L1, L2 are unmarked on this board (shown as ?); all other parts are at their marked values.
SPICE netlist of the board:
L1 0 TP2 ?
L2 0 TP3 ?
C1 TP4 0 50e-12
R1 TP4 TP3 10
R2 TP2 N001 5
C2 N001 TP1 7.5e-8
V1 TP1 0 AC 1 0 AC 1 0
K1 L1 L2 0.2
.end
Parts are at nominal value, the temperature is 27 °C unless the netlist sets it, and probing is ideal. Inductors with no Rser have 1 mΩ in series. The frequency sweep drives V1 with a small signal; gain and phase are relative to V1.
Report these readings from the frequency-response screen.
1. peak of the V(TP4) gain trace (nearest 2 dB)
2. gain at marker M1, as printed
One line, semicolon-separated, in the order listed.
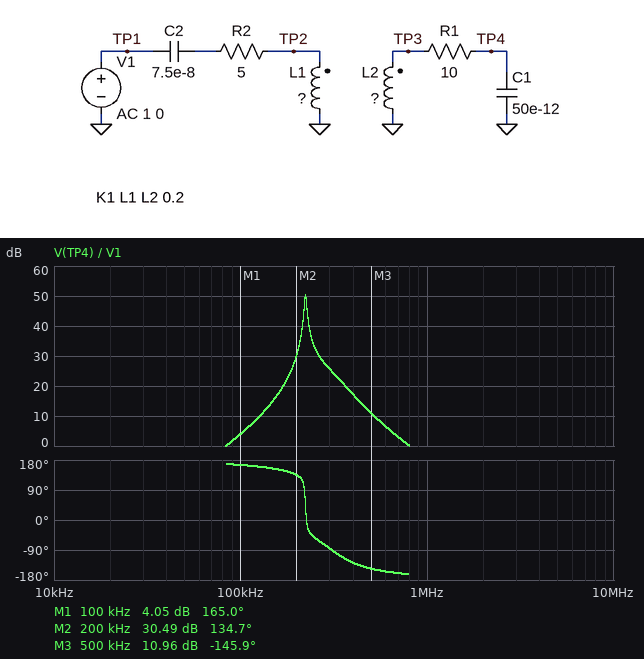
50 dB; 4.05 dB
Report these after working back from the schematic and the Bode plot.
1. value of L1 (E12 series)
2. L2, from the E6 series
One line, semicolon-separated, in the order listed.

3.9 µH; 10 mH
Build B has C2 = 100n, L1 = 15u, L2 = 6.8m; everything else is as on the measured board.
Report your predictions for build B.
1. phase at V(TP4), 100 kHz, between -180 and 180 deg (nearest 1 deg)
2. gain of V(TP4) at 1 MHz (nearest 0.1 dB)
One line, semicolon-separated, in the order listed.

142 deg; -8.8 dB
